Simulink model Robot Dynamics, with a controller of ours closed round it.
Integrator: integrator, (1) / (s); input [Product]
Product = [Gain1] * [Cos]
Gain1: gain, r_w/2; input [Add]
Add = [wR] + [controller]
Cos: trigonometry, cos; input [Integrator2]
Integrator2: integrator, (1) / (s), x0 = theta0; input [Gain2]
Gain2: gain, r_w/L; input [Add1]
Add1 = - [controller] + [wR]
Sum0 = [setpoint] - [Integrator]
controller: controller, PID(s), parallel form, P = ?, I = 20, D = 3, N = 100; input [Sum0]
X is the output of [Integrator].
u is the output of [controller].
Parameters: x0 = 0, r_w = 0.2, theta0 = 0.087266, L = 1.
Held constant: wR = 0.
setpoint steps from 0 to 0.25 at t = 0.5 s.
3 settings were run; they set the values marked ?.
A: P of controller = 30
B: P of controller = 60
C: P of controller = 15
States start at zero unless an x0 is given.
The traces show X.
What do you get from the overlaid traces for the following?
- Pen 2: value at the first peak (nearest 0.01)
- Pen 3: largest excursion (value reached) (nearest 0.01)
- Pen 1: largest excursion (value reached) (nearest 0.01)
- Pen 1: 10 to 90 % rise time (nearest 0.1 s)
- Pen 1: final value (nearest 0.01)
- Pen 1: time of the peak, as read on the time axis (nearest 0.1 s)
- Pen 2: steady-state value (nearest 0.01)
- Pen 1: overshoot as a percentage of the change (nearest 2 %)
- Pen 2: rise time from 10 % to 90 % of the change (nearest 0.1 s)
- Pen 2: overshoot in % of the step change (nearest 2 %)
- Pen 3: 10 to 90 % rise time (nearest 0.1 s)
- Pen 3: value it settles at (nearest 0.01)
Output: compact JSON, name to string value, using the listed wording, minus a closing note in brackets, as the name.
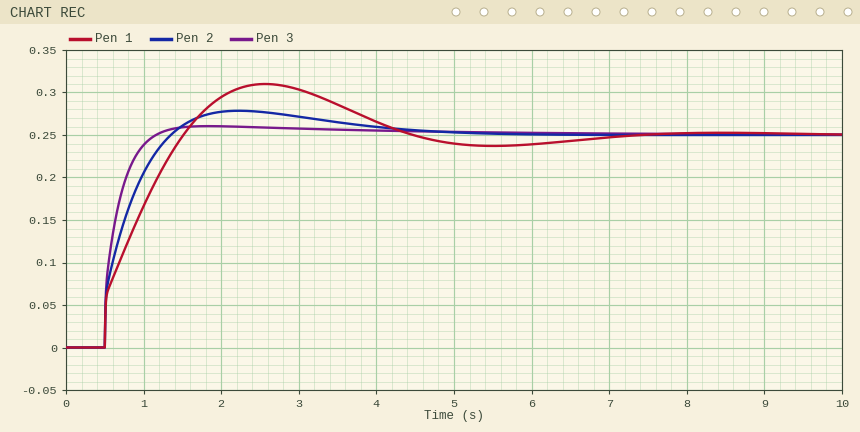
{"Pen 2: value at the first peak": "0.28", "Pen 3: largest excursion (value reached)": "0.26", "Pen 1: largest excursion (value reached)": "0.31", "Pen 1: 10 to 90 % rise time": "0.8 s", "Pen 1: final value": "0.25", "Pen 1: time of the peak, as read on the time axis": "2.6 s", "Pen 2: steady-state value": "0.25", "Pen 1: overshoot as a percentage of the change": "24 %", "Pen 2: rise time from 10 % to 90 % of the change": "0.6 s", "Pen 2: overshoot in % of the step change": "12 %", "Pen 3: 10 to 90 % rise time": "0.4 s", "Pen 3: value it settles at": "0.25"}
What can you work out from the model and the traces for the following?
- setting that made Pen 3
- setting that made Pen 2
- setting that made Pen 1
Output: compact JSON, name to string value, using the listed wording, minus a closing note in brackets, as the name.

{"setting that made Pen 3": "B", "setting that made Pen 2": "A", "setting that made Pen 1": "C"}
